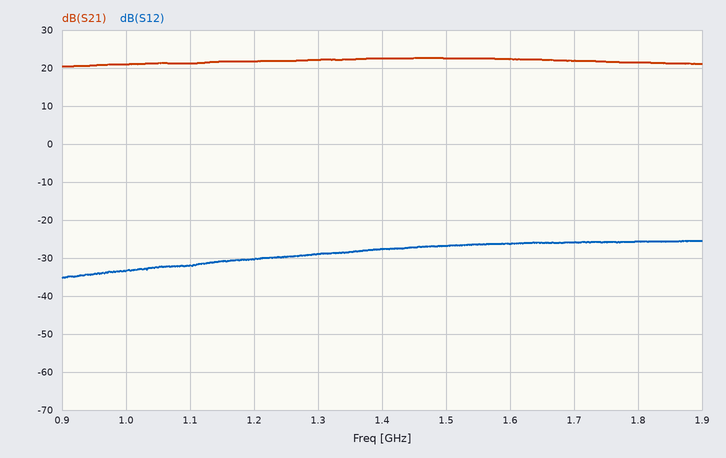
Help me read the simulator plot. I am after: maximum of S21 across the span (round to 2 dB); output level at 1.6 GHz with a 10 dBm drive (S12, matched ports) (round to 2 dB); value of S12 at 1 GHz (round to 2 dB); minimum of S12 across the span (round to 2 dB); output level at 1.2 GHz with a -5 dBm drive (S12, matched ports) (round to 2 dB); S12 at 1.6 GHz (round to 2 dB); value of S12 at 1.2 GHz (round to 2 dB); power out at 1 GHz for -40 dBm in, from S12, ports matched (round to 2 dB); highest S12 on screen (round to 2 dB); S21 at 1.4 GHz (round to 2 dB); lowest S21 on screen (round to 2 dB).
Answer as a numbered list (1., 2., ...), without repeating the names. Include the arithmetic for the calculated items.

1. 22 dB
2. 10 dBm + (-26 dB) = -16 dBm
3. -34 dB
4. -36 dB
5. -5 dBm + (-30 dB) = -36 dBm
6. -26 dB
7. -30 dB
8. -40 dBm + (-34 dB) = -74 dBm
9. -26 dB
10. 22 dB
11. 20 dB
